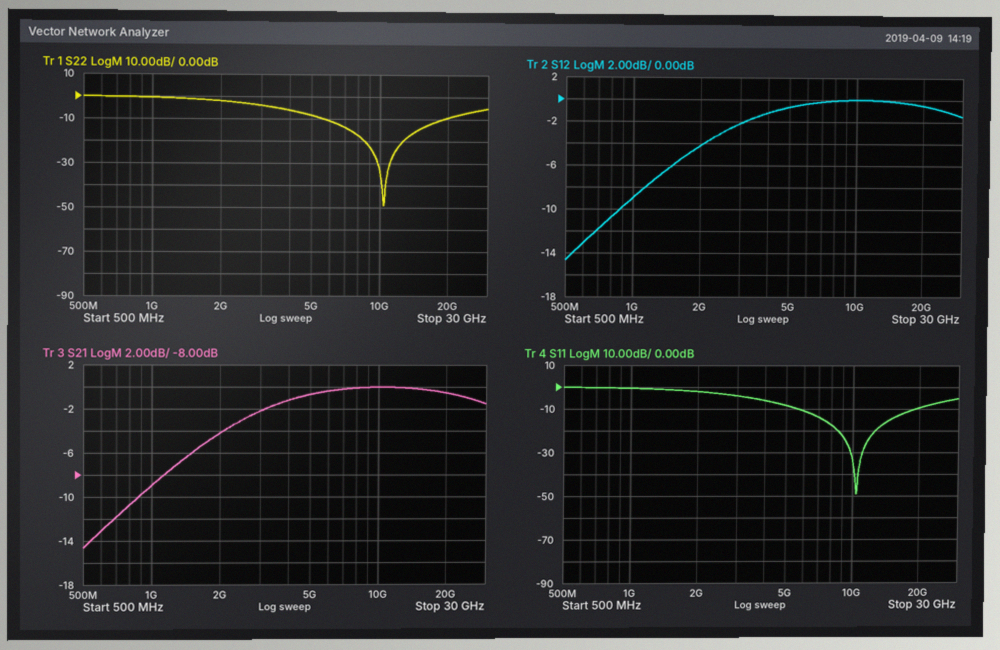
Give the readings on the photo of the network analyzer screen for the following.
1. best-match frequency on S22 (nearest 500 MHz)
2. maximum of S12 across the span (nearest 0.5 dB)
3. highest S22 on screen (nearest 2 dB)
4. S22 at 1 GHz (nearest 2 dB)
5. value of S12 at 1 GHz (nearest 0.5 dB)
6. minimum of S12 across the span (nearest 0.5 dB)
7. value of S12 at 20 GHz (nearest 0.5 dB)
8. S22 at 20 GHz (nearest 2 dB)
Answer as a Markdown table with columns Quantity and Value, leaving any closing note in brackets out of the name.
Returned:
| Quantity | Value |
|---|---|
| best-match frequency on S22 | 10.5 GHz |
| maximum of S12 across the span | 0.0 dB |
| highest S22 on screen | 0 dB |
| S22 at 1 GHz | 0 dB |
| value of S12 at 1 GHz | -9.0 dB |
| minimum of S12 across the span | -14.5 dB |
| value of S12 at 20 GHz | -0.5 dB |
| S22 at 20 GHz | -10 dB |
